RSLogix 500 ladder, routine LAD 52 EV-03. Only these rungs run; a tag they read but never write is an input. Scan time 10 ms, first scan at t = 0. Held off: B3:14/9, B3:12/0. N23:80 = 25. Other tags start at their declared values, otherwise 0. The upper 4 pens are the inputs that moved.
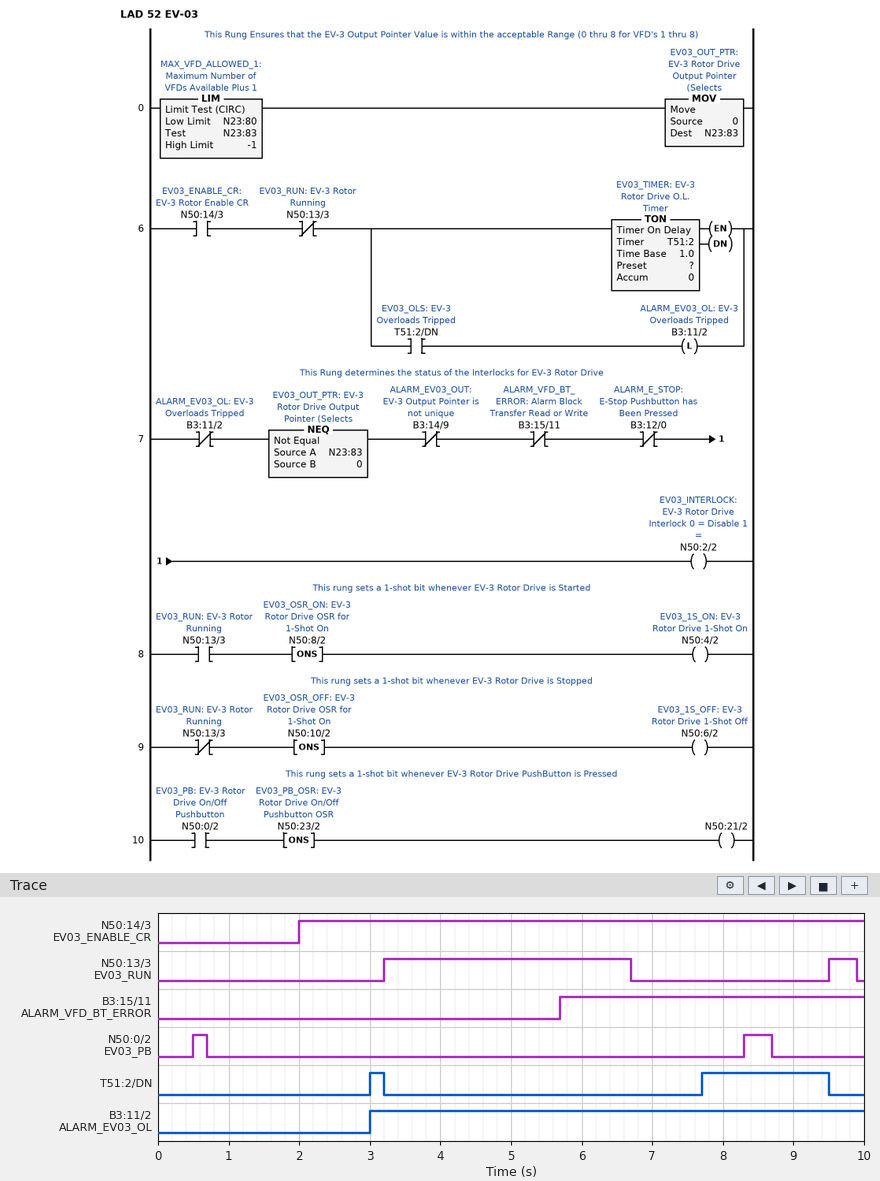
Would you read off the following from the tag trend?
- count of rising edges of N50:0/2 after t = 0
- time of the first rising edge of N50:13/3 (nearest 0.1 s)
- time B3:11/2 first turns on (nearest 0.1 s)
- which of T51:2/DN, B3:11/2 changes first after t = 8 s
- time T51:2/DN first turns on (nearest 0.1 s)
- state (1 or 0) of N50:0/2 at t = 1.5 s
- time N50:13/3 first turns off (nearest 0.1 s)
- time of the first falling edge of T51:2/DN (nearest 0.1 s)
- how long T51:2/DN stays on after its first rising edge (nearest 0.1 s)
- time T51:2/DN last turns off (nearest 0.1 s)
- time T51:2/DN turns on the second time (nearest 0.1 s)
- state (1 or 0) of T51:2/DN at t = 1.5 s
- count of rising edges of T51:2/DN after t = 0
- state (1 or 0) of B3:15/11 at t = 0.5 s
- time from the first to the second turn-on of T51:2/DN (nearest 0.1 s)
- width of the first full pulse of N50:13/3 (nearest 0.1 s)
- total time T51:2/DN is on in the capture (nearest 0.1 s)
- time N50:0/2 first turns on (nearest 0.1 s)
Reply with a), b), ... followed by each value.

a) 2
b) 3.2 s
c) 3.0 s
d) T51:2/DN
e) 3.0 s
f) 0
g) 6.7 s
h) 3.2 s
i) 0.2 s
j) 9.5 s
k) 7.7 s
l) 0
m) 2
n) 0
o) 4.7 s
p) 3.5 s
q) 2.0 s
r) 0.5 s
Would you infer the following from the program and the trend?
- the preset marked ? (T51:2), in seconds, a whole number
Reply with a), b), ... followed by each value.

a) 1 s
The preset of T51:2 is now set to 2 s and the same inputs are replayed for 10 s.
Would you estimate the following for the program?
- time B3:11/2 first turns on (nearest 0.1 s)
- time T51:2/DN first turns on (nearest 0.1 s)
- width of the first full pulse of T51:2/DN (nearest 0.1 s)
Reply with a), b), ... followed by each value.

a) 8.7 s
b) 8.7 s
c) 0.8 s
